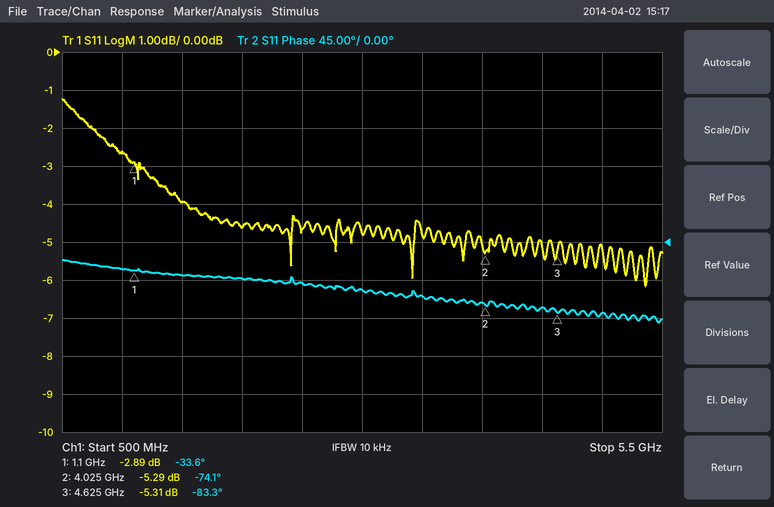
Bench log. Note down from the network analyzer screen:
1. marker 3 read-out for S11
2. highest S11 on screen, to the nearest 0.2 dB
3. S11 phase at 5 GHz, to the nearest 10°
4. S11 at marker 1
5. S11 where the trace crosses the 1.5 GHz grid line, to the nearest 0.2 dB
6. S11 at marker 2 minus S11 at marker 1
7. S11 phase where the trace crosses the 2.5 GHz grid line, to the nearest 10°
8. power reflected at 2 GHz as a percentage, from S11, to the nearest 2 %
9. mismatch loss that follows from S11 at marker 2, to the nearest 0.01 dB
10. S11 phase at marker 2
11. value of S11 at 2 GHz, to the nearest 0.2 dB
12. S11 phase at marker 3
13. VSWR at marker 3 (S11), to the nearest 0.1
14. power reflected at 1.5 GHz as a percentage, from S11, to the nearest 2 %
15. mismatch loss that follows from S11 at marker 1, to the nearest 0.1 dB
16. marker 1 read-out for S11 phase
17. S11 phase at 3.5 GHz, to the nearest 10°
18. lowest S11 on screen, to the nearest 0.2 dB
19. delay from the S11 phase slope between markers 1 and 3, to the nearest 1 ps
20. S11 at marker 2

-5.31 dB
-1.2 dB
-80°
-2.89 dB
-4.0 dB
-2.40 dB
-50°
34 %
1.52 dB
-74.1°
-4.6 dB
-83.3°
3.4
40 %
3.1 dB
-33.6°
-60°
-6.2 dB
39 ps
-5.29 dB
